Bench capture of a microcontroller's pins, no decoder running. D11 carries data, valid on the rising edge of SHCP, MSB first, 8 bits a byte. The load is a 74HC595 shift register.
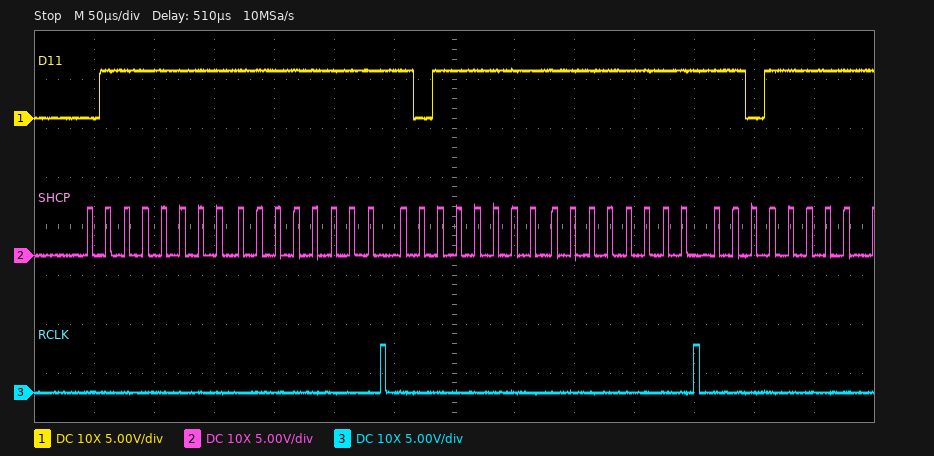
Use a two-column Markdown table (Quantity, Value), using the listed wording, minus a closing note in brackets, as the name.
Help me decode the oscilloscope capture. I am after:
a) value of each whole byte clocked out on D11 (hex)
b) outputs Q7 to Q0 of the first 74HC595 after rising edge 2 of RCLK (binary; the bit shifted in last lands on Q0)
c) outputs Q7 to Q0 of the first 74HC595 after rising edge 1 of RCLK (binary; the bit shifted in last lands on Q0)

| Quantity | Value |
|---|---|
| value of each whole byte clocked out on D11 | 7F FF BF FF DF |
| outputs Q7 to Q0 of the first 74HC595 after rising edge 2 of RCLK | 11111111 |
| outputs Q7 to Q0 of the first 74HC595 after rising edge 1 of RCLK | 11111111 |
